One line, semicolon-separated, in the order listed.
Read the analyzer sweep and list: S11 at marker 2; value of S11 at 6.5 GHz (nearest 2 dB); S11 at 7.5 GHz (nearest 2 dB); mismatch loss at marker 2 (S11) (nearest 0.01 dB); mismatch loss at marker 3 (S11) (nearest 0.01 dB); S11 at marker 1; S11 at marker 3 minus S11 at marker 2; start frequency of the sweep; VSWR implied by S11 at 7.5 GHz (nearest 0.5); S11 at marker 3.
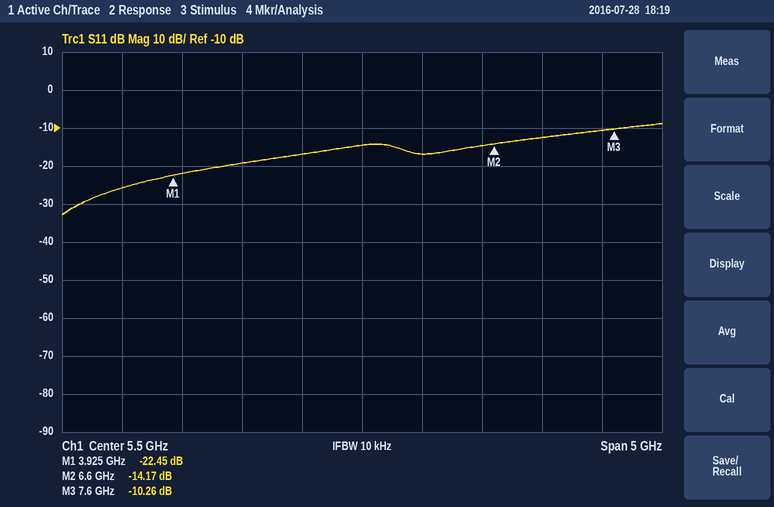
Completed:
-14.17 dB; -14 dB; -10 dB; 0.17 dB; 0.43 dB; -22.45 dB; 3.91 dB; 3 GHz; 2.0; -10.26 dB
